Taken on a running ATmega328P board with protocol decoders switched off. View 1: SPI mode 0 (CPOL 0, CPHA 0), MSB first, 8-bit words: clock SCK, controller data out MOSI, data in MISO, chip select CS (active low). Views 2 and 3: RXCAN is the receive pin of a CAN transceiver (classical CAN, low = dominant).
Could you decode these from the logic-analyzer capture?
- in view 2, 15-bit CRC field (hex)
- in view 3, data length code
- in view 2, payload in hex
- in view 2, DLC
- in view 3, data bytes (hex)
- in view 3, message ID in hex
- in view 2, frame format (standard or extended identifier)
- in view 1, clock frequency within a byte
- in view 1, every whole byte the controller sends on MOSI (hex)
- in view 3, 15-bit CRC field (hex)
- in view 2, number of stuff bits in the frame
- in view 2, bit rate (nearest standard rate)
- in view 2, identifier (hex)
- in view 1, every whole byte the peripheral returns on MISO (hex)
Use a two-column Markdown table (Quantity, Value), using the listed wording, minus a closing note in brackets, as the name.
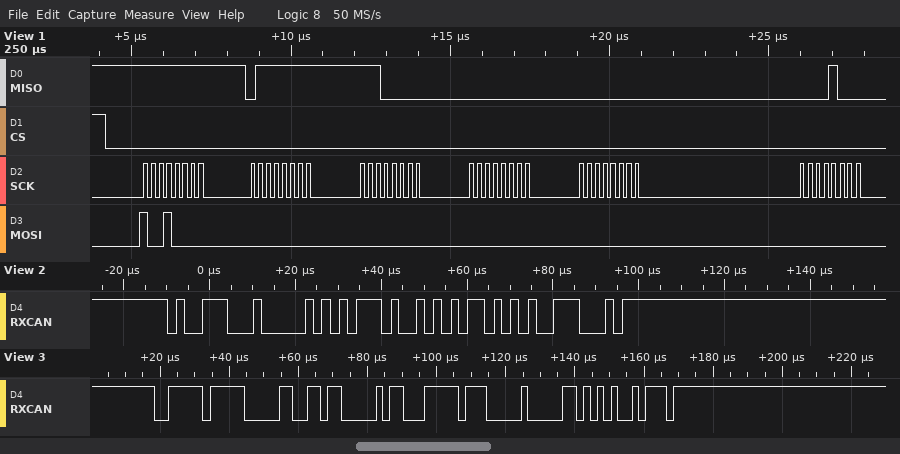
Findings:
| Quantity | Value |
|---|---|
| in view 2, 15-bit CRC field | 0x5538 |
| in view 3, data length code | 4 |
| in view 2, payload in hex | BA 55 |
| in view 2, DLC | 2 |
| in view 3, data bytes | D8 18 FF 00 |
| in view 3, message ID in hex | 0x3FF |
| in view 2, frame format | standard |
| in view 1, clock frequency within a byte | 4 MHz |
| in view 1, every whole byte the controller sends on MOSI | 0x90 0x00 0x00 0x00 0x00 0x00 |
| in view 3, 15-bit CRC field | 0x154B |
| in view 2, number of stuff bits in the frame | 1 |
| in view 2, bit rate | 500 kbit/s |
| in view 2, identifier | 0x4E2 |
| in view 1, every whole byte the peripheral returns on MISO | 0xFF 0x7F 0xE0 0x00 0x00 0x08 |
